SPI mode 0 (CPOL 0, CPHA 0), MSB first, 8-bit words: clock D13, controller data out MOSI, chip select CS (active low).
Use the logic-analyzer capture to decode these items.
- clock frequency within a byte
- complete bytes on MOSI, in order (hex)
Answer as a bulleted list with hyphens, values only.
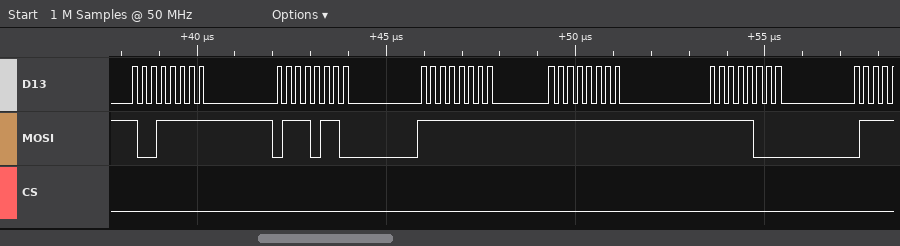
- 4 MHz
- 9F 76 FF FF F8
